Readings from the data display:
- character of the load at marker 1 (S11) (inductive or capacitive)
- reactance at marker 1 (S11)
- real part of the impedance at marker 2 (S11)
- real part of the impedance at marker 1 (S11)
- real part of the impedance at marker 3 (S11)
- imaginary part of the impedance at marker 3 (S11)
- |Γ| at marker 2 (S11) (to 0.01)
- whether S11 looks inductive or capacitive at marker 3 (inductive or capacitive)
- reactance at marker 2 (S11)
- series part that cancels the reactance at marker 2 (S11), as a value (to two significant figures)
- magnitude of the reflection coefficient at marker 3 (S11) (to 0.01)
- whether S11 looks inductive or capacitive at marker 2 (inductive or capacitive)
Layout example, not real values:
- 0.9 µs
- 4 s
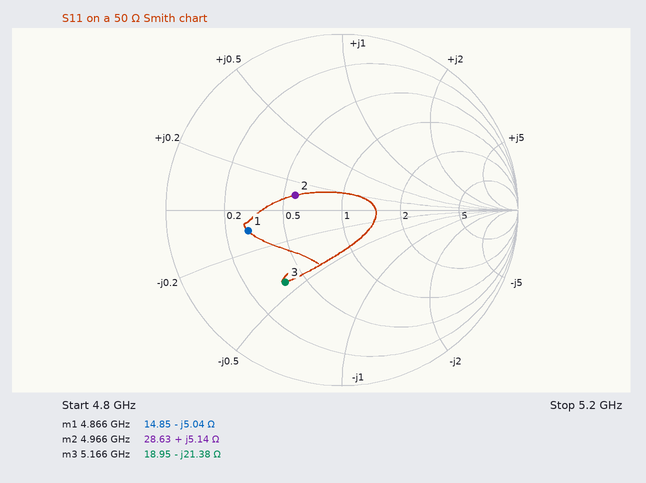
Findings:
- capacitive
- -5.04 Ω
- 28.63 Ω
- 14.85 Ω
- 18.95 Ω
- -21.38 Ω
- 0.28
- capacitive
- +5.14 Ω
- 6.2 pF
- 0.52
- inductive
